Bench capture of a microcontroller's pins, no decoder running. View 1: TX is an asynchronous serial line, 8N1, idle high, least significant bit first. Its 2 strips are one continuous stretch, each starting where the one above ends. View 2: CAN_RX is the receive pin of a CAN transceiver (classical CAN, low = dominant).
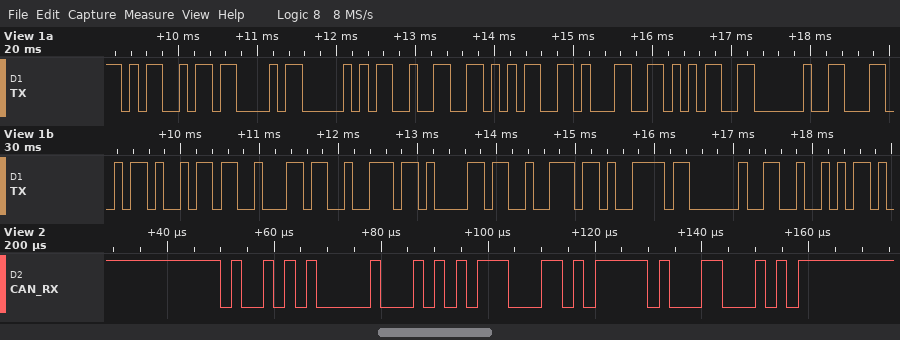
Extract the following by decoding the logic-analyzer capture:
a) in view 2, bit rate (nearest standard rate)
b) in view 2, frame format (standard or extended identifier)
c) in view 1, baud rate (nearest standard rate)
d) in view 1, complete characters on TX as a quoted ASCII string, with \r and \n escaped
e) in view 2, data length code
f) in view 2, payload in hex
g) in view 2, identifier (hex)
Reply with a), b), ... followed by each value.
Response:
a) 500 kbit/s
b) standard
c) 9600 baud
d) "MCP2515 Library R"
e) 2
f) AE 35
g) 0x4A8
